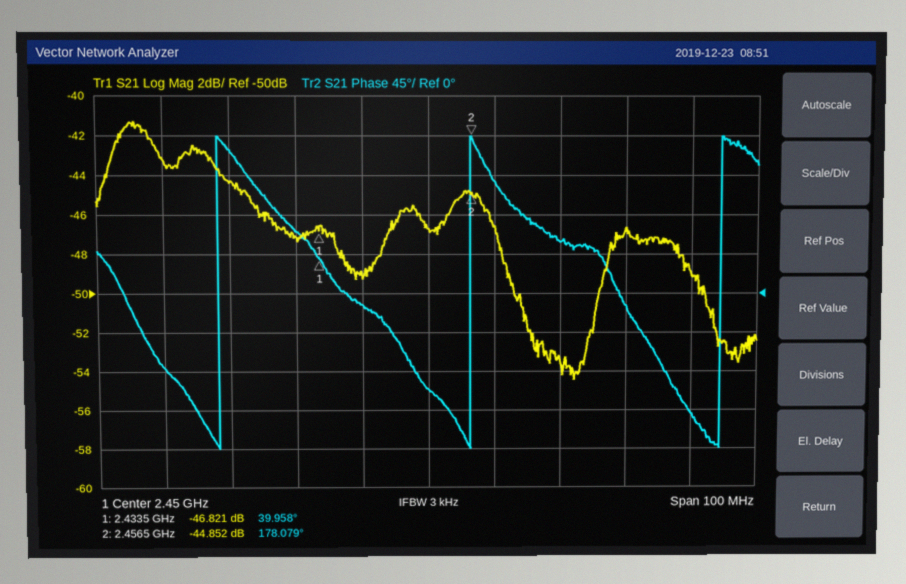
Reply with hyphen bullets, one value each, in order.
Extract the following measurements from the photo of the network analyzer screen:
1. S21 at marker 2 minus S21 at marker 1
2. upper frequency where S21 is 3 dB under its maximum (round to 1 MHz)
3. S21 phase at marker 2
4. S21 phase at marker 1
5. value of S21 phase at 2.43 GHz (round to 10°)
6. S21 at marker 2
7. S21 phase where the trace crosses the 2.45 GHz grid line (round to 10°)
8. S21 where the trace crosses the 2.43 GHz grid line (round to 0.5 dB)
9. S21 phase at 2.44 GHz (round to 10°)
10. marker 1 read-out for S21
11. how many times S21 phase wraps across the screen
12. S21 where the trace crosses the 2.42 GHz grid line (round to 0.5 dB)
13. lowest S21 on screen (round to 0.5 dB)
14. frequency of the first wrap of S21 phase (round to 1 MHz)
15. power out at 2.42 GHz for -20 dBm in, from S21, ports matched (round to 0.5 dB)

- 1.969 dB
- 2.420 GHz
- 178.079°
- 39.958°
- 70°
- -44.852 dB
- -110°
- -47.0 dB
- -10°
- -46.821 dB
- 3
- -44.5 dB
- -54.5 dB
- 2.418 GHz
- -64.5 dBm
